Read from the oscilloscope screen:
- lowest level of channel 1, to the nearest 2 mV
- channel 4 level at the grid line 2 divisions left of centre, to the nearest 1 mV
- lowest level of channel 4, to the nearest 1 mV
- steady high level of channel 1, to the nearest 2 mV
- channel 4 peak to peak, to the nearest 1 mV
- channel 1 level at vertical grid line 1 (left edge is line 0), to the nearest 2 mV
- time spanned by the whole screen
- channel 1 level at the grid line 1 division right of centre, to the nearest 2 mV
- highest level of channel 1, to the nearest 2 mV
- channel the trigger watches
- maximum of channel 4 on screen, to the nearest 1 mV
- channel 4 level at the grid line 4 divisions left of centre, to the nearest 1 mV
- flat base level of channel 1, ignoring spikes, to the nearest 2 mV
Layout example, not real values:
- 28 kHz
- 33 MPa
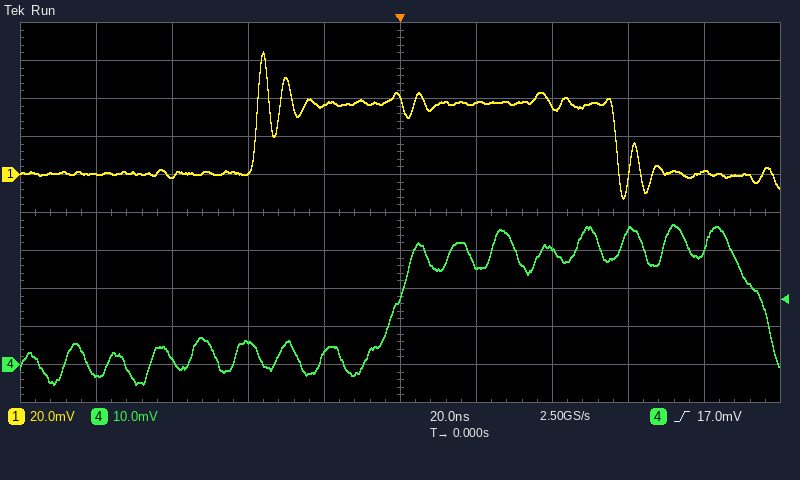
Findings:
- -12 mV
- 6 mV
- -5 mV
- 38 mV
- 42 mV
- 0 mV
- 200 ns
- 38 mV
- 64 mV
- channel 4
- 37 mV
- -3 mV
- 0 mV
